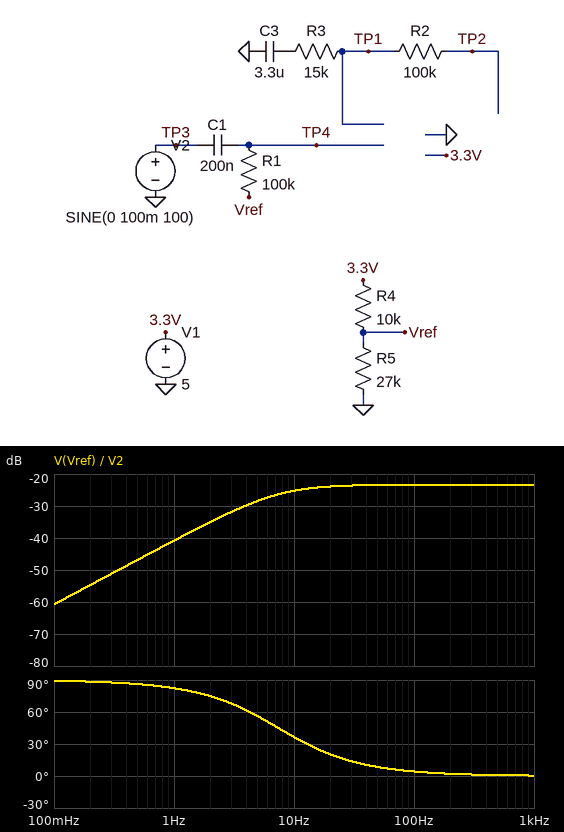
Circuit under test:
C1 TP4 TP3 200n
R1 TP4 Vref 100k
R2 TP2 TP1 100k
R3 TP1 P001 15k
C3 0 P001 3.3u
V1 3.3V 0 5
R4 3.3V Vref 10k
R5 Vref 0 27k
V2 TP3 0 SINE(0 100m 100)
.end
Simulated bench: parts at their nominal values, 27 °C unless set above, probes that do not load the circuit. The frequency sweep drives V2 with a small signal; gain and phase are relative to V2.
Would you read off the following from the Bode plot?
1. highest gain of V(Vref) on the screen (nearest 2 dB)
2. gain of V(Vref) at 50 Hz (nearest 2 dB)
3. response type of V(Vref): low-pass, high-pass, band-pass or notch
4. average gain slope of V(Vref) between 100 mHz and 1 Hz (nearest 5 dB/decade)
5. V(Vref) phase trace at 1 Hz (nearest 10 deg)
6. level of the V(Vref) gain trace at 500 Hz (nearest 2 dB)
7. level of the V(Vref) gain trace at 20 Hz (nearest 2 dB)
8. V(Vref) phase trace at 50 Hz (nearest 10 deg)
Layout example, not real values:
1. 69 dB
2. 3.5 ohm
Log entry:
1. -24 dB
2. -24 dB
3. high-pass
4. 20 dB/decade
5. 80 deg
6. -24 dB
7. -24 dB
8. 10 deg
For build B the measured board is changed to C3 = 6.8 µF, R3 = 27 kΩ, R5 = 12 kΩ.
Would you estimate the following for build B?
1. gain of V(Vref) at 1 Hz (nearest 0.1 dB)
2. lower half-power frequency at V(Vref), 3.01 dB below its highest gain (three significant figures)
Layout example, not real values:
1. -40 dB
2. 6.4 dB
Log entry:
1. -43.4 dB
2. 7.55 Hz
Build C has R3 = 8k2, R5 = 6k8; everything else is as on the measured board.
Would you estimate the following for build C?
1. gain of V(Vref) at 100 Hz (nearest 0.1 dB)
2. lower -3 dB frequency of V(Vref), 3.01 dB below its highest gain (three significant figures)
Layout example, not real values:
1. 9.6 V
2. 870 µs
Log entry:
1. -28.2 dB
2. 7.65 Hz
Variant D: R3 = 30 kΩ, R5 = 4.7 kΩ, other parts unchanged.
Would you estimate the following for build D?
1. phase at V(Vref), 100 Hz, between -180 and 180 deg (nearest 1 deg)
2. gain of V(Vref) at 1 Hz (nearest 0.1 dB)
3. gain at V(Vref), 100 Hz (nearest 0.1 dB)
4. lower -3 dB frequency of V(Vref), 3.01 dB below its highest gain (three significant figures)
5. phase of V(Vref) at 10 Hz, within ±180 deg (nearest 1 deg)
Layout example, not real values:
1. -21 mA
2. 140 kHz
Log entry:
1. 4 deg
2. -48.0 dB
3. -30.2 dB
4. 7.71 Hz
5. 38 deg
